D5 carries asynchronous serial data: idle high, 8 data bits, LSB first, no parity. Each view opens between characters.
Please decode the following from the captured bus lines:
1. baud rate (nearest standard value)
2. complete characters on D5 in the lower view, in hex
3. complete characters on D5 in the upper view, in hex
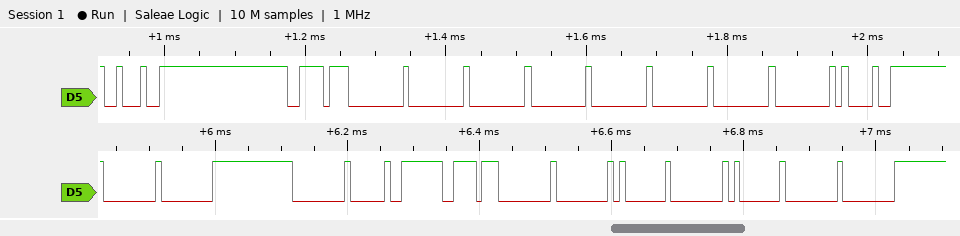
115200 baud
00, 00, 00, 20, DE, 00, 00, 01, 00, 01, 00, 00
22, DE, 00, 00, 00, 00, 00, 00, 00, 00, 21
